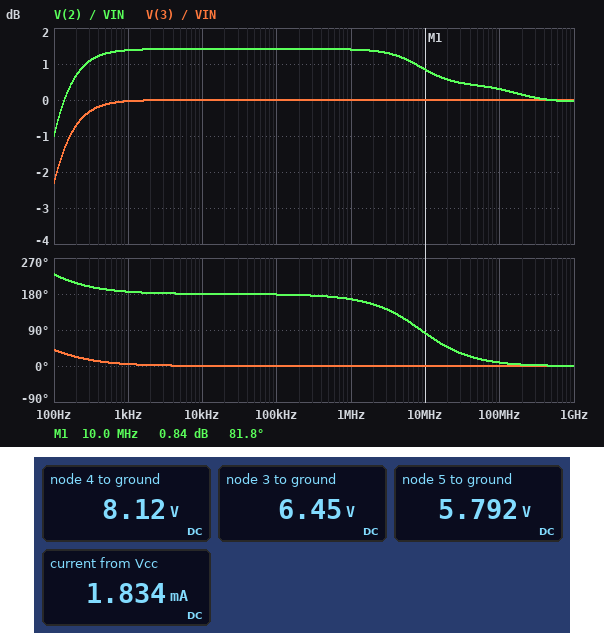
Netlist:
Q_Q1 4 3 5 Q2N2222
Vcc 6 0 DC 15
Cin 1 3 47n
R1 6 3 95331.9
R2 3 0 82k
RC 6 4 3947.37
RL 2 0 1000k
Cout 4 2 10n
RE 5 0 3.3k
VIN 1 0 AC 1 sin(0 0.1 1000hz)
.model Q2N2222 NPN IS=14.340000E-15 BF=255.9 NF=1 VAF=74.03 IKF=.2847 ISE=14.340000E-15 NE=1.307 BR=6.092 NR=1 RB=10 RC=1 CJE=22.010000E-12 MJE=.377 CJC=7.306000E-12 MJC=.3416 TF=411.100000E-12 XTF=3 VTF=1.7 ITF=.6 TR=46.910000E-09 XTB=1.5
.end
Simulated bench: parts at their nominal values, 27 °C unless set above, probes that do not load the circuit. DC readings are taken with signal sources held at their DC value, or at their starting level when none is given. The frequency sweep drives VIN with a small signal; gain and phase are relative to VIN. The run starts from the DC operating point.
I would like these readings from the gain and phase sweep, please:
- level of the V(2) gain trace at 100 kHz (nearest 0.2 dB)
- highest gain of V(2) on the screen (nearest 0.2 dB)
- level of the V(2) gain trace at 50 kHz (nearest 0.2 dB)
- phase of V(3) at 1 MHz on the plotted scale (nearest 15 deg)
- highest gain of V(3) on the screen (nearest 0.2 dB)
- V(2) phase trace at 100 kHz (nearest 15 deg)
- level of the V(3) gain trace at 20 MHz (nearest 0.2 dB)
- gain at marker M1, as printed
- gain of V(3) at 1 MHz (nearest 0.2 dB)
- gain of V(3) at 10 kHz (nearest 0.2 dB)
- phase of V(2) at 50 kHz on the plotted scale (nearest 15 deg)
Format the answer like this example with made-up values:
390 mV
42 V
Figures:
1.4 dB
1.4 dB
1.4 dB
0 deg
0 dB
180 deg
0 dB
0.84 dB
0 dB
0 dB
180 deg
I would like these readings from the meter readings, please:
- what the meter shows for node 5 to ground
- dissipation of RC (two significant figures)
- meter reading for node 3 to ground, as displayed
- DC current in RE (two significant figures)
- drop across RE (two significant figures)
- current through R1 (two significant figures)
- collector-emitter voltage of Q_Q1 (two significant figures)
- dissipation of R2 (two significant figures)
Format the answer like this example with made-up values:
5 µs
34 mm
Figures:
5.792 V
12 mW
6.45 V
1.8 mA
5.8 V
90 µA
2.3 V
510 µW
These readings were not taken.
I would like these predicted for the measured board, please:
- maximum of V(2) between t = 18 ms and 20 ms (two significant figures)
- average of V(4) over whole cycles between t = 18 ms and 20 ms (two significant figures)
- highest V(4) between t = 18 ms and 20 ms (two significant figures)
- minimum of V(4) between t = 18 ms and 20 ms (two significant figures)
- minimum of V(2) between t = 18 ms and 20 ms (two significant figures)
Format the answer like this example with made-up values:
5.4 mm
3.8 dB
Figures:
120 mV
8.1 V
8.2 V
8.0 V
-120 mV
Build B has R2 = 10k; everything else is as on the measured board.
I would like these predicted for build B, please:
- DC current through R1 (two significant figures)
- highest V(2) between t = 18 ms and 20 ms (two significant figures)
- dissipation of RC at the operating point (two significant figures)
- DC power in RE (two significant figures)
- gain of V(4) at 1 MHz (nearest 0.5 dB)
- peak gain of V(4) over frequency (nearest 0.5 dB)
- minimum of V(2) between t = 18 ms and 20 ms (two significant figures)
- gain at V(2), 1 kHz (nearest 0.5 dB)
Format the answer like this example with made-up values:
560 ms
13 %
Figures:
140 µA
110 mV
230 µW
200 µW
1.0 dB
1.5 dB
-110 mV
0.5 dB
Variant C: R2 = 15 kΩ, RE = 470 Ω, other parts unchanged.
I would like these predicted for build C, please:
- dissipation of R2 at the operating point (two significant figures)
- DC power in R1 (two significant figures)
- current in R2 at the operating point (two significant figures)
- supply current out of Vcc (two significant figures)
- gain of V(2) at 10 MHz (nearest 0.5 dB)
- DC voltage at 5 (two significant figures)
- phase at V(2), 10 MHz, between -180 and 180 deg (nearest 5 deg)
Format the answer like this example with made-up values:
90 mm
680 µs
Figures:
230 µW
1.8 mW
120 µA
2.6 mA
15.0 dB
1.2 V
125 deg
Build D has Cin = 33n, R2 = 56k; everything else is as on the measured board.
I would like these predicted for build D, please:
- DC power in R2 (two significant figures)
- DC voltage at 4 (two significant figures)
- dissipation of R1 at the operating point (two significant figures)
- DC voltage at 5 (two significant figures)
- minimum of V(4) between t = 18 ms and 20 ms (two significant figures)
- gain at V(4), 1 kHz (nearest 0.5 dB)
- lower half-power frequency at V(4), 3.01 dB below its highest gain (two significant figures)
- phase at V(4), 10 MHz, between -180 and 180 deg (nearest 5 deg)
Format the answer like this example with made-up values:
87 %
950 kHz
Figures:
490 µW
9.5 V
1.0 mW
4.6 V
9.4 V
1.5 dB
150 Hz
95 deg
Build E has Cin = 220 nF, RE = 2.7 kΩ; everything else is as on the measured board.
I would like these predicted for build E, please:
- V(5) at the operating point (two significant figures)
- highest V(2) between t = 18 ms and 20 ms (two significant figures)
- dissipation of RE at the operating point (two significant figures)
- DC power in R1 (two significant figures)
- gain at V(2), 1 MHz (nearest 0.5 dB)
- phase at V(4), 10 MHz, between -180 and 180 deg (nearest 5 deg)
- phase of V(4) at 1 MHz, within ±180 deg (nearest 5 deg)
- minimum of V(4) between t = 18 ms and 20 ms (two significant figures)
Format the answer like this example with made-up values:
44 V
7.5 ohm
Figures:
5.7 V
140 mV
12 mW
780 µW
3.0 dB
75 deg
165 deg
6.6 V
